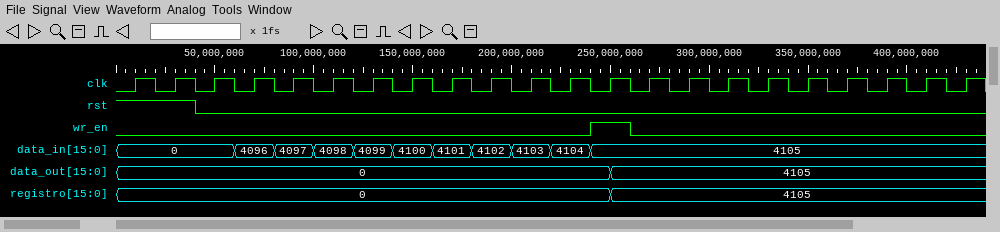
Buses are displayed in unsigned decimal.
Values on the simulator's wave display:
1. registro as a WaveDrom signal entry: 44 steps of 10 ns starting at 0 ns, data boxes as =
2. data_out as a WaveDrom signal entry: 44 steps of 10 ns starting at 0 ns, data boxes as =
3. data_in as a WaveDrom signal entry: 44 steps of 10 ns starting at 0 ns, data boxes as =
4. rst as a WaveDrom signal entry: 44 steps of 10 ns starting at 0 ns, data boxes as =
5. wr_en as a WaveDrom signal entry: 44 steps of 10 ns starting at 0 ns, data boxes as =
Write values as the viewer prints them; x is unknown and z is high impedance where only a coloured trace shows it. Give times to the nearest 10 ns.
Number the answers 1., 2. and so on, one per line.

1. {name: 'registro', wave: '=........................=..................', data: '0 4105'}
2. {name: 'data_out', wave: '=........................=..................', data: '0 4105'}
3. {name: 'data_in', wave: '=.....=.=.=.=.=.=.=.=.=.=...................', data: '0 4096 4097 4098 4099 4100 4101 4102 4103 4104 4105'}
4. {name: 'rst', wave: '1...0.......................................'}
5. {name: 'wr_en', wave: '0.......................1.0.................'}
